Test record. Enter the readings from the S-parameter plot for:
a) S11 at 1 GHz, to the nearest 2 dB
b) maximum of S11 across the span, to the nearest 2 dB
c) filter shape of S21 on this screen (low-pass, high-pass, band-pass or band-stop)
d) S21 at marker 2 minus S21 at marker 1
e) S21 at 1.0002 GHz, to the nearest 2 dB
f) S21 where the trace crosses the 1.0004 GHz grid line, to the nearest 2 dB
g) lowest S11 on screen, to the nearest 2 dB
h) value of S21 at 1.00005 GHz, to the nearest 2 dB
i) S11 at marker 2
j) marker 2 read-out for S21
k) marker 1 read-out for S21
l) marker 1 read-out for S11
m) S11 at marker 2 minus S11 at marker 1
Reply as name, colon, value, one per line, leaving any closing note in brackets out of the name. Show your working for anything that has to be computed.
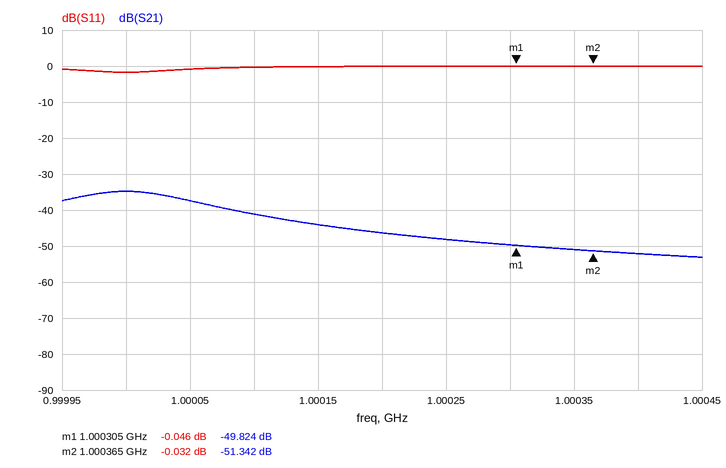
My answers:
S11 at 1 GHz, to the nearest 2 dB: -2 dB
maximum of S11 across the span, to the nearest 2 dB: 0 dB
filter shape of S21 on this screen: low-pass
S21 at marker 2 minus S21 at marker 1: -51.342 − (-49.824) = -1.518 dB
S21 at 1.0002 GHz, to the nearest 2 dB: -46 dB
S21 where the trace crosses the 1.0004 GHz grid line, to the nearest 2 dB: -52 dB
lowest S11 on screen, to the nearest 2 dB: -2 dB
value of S21 at 1.00005 GHz, to the nearest 2 dB: -38 dB
S11 at marker 2: -0.032 dB
marker 2 read-out for S21: -51.342 dB
marker 1 read-out for S21: -49.824 dB
marker 1 read-out for S11: -0.046 dB
S11 at marker 2 minus S11 at marker 1: -0.032 − (-0.046) = 0.014 dB
